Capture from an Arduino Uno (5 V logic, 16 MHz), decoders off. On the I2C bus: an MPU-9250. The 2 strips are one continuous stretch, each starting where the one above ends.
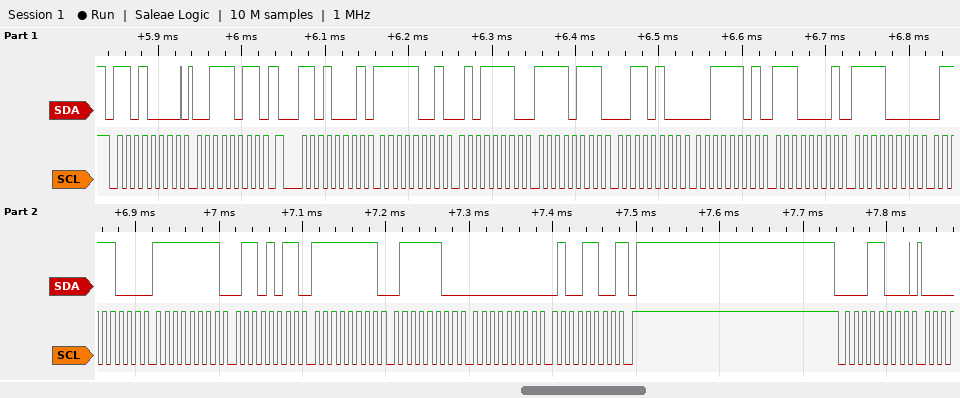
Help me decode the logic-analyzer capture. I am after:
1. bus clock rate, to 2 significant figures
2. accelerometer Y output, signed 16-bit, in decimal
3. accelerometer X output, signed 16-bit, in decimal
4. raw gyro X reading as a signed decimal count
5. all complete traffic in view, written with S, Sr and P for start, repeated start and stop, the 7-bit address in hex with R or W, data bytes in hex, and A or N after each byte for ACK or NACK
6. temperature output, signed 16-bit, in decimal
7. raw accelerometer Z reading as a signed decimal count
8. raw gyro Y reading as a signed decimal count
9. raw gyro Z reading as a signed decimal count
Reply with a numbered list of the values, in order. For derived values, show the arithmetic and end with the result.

1. 100 kHz
2. 0xF734 = -2252
3. 0xF95E = -1698
4. 0xFF6B = -149
5. S 68W A 3B A Sr 68R A F9 A 5E A F7 A 34 A 3D A E1 A F0 A 78 A FF A 6B A FF A 7C A 00 A 4C N P S 0CW A
6. 0xF078 = -3976
7. 0x3DE1 = 15841
8. 0xFF7C = -132
9. 0x004C = 76
